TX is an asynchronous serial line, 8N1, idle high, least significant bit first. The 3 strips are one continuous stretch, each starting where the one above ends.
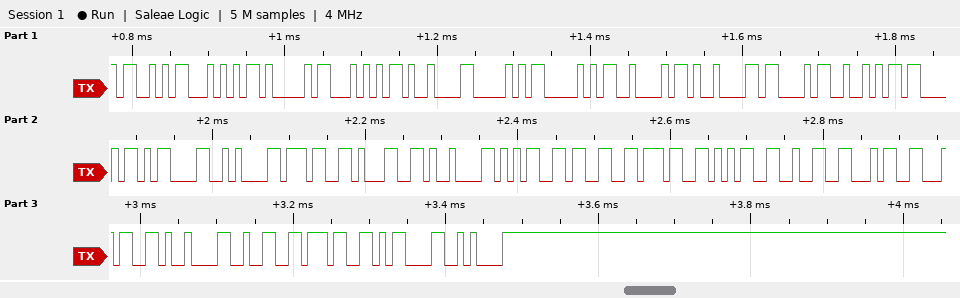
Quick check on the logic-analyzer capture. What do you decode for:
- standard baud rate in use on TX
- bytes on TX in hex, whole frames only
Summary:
115200 baud
53 54 41 54 09 50 50 42 09 43 52 43 0D 0A 37 31 09 35 33 37 35 32 34 34 09 32 37 0D 0A
